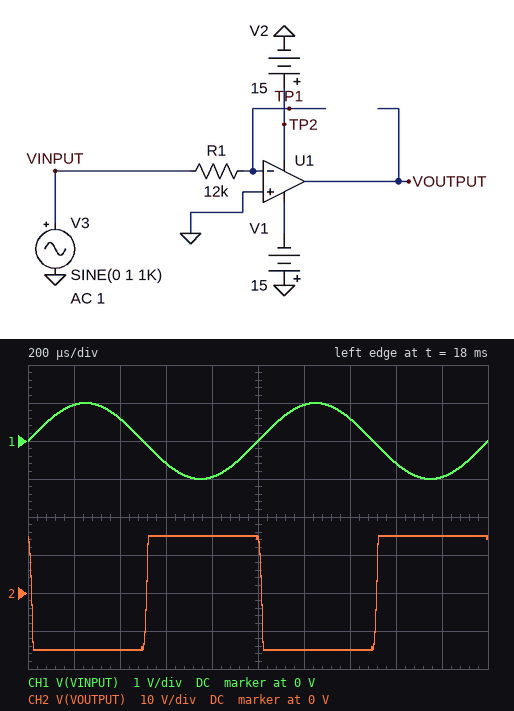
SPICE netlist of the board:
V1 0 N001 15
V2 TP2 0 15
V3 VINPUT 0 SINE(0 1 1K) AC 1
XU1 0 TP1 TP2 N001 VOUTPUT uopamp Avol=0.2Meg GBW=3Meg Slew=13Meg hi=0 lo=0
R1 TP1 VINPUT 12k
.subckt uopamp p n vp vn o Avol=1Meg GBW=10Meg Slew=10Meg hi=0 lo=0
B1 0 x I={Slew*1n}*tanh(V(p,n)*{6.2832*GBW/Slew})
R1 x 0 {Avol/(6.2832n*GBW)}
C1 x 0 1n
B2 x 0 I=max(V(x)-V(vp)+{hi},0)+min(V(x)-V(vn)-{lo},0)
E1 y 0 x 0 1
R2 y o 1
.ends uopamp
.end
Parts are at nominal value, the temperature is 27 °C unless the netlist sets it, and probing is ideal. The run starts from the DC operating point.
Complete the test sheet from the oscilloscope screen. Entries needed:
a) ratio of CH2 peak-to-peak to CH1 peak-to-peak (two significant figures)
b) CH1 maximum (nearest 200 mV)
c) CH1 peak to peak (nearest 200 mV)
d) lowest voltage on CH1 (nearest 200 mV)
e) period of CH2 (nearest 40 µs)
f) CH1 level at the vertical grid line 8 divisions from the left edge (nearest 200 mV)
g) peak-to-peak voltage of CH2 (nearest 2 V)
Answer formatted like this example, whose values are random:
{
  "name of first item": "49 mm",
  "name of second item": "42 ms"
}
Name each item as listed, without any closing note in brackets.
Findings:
{
  "ratio of CH2 peak-to-peak to CH1 peak-to-peak": "15",
  "CH1 maximum": "1.0 V",
  "CH1 peak to peak": "2.0 V",
  "lowest voltage on CH1": "-1.0 V",
  "period of CH2": "1.00 ms",
  "CH1 level at the vertical grid line 8 divisions from the left edge": "-600 mV",
  "peak-to-peak voltage of CH2": "30 V"
}
